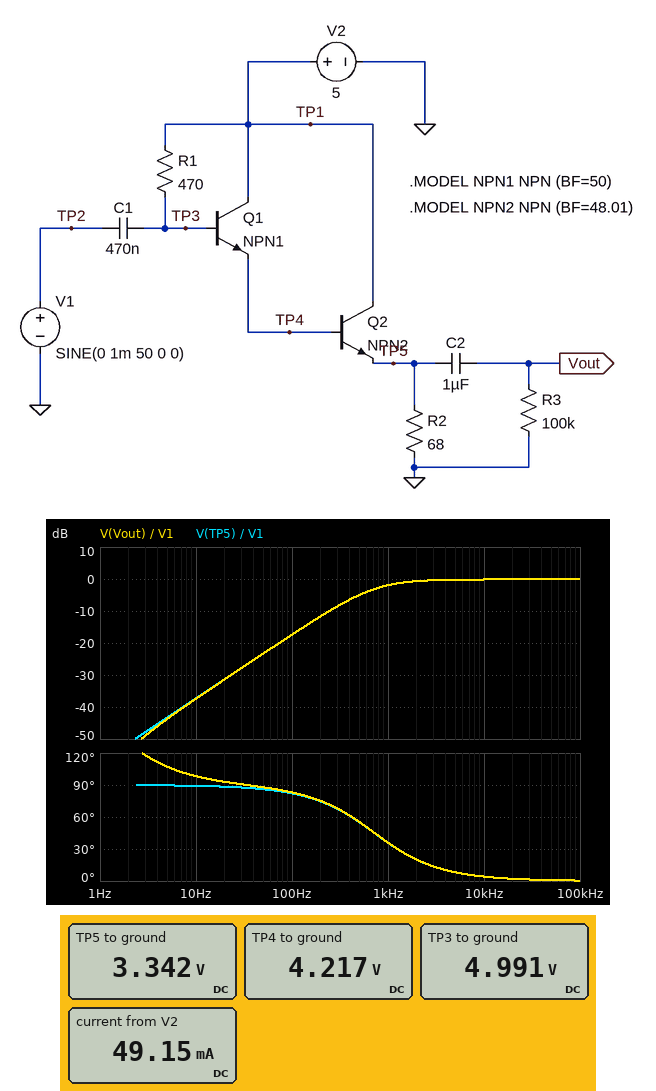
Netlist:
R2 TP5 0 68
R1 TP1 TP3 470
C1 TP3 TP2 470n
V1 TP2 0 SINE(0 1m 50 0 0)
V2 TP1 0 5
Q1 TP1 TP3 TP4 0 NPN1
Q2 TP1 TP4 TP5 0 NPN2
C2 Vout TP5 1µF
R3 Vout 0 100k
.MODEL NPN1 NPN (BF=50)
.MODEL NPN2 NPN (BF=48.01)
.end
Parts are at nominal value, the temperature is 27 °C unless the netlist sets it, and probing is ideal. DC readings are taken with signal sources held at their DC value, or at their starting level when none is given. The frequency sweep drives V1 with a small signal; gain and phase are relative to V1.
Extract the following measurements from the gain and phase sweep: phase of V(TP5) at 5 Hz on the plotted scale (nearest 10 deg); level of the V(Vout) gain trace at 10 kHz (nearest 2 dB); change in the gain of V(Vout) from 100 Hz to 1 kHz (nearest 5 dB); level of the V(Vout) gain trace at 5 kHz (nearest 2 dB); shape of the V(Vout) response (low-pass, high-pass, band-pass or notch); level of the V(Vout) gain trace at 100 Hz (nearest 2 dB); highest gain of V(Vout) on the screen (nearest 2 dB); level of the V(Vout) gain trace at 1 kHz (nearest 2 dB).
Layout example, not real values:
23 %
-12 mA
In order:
90 deg
0 dB
15 dB
0 dB
high-pass
-18 dB
0 dB
-2 dB
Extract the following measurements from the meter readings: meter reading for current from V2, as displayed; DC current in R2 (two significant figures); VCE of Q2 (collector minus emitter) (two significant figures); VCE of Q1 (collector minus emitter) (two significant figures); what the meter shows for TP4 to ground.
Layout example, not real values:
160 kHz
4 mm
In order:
49.15 mA
49 mA
1.7 V
780 mV
4.217 V
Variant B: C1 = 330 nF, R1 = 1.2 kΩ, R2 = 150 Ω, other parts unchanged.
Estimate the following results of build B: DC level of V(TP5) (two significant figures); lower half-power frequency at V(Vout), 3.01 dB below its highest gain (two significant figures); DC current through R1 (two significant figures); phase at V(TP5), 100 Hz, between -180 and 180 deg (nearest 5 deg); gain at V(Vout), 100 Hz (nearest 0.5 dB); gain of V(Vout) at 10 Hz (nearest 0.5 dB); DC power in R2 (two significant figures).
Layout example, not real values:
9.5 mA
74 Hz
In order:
3.4 V
400 Hz
9.0 µA
75 deg
-12.5 dB
-32.5 dB
76 mW
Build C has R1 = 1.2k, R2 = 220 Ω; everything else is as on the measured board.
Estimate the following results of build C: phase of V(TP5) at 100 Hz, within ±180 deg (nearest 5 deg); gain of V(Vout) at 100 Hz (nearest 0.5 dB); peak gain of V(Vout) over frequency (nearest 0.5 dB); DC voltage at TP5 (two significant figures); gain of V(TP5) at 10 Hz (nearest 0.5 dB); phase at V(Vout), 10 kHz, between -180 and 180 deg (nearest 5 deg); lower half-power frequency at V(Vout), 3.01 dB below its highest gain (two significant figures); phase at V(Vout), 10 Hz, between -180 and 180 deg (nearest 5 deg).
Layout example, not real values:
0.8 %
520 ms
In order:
70 deg
-9.5 dB
0 dB
3.4 V
-29.0 dB
0 deg
280 Hz
95 deg
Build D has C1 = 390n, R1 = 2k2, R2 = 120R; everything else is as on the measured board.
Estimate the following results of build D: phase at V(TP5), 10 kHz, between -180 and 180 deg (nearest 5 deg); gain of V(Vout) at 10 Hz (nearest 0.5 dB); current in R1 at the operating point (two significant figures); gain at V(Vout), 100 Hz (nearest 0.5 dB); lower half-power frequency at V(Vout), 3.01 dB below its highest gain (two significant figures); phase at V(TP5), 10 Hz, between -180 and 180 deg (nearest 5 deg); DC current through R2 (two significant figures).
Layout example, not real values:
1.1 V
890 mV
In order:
0 deg
-25.5 dB
11 µA
-6.5 dB
190 Hz
85 deg
28 mA
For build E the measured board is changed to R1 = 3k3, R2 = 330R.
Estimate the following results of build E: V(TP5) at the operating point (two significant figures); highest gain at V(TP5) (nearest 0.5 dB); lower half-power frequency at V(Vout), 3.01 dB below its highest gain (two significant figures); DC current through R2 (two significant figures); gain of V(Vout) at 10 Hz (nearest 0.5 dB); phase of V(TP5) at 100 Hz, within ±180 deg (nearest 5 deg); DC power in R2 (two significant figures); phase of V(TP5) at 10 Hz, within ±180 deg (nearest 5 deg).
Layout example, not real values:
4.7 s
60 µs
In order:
3.4 V
0 dB
100 Hz
10 mA
-20.5 dB
45 deg
35 mW
85 deg
